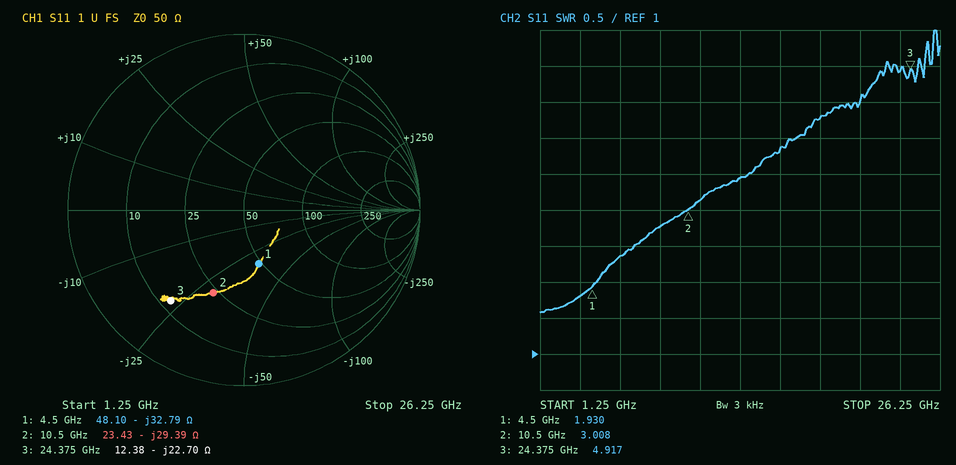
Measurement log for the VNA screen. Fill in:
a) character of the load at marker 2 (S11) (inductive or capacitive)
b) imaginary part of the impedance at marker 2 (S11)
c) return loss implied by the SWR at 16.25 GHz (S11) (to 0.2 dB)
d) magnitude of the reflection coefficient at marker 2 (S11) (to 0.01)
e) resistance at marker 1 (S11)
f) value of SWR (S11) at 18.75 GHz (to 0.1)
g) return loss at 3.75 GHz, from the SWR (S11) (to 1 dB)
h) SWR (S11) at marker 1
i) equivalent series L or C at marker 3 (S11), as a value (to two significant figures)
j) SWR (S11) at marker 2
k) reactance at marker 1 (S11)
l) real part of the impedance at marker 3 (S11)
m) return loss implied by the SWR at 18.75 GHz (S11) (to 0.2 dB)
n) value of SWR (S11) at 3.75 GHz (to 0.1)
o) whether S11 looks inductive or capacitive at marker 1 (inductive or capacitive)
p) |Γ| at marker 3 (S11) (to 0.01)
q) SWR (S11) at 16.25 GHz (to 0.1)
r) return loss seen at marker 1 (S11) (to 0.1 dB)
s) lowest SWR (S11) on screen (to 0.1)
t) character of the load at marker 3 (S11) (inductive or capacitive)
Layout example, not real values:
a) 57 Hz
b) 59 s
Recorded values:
a) capacitive
b) -29.39 Ω
c) 4.6 dB
d) 0.50
e) 48.10 Ω
f) 4.3
g) 11 dB
h) 1.930
i) 290 fF
j) 3.008
k) -32.79 Ω
l) 12.38 Ω
m) 4.2 dB
n) 1.8
o) capacitive
p) 0.66
q) 3.8
r) 10.0 dB
s) 1.6
t) capacitive
